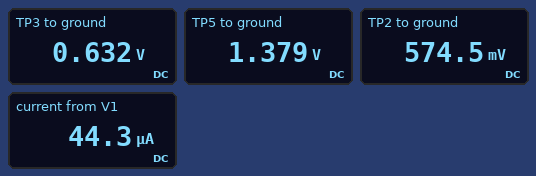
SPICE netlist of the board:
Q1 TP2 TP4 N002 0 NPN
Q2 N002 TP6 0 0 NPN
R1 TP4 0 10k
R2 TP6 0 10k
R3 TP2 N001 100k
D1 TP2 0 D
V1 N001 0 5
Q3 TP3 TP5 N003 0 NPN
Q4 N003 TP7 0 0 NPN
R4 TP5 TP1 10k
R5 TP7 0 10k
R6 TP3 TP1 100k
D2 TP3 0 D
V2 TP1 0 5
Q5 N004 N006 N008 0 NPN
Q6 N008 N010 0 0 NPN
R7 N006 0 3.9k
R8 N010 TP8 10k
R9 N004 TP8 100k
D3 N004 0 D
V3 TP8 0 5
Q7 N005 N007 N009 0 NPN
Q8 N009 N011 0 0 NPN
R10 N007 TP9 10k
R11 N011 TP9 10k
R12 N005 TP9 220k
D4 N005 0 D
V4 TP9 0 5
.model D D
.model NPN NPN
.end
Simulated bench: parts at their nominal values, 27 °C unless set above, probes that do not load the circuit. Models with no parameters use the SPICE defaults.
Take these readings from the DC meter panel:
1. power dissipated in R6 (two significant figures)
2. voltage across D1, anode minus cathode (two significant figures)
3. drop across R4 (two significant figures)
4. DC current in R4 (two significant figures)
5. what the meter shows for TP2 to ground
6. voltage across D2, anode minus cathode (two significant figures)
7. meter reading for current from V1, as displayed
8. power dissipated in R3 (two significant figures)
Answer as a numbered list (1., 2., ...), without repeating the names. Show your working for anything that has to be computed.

1. (5 V - 632 mV)^2 / 100 kΩ = 190 µW
2. 574.5 mV = 570 mV
3. 5 V - 1.379 V = 3.6 V
4. (5 V - 1.379 V) / 10 kΩ = 360 µA
5. 574.5 mV
6. 632 mV = 630 mV
7. 44.3 µA
8. (5 V - 574.5 mV)^2 / 100 kΩ = 200 µW
